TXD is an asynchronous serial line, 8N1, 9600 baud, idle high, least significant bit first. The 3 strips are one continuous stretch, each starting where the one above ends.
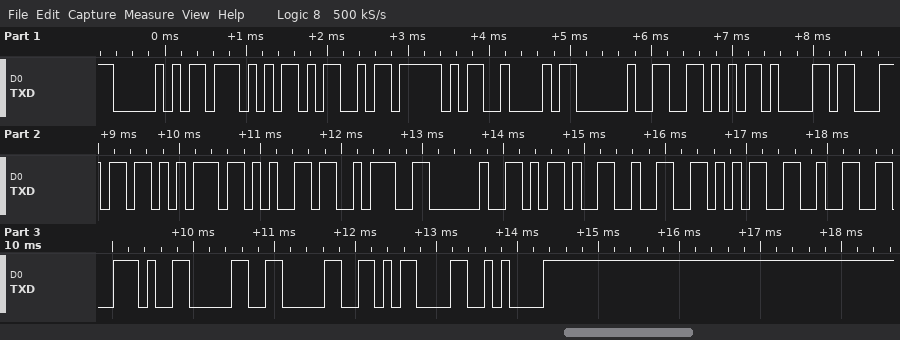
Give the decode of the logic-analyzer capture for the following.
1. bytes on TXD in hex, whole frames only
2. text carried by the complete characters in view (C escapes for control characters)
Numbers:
50 57 4D 5F 42 20 56 61 6C 75 65 3A 20 2D 32 35 32 2E 30 30 0D 0A
"PWM_B Value: -252.00\r\n"
